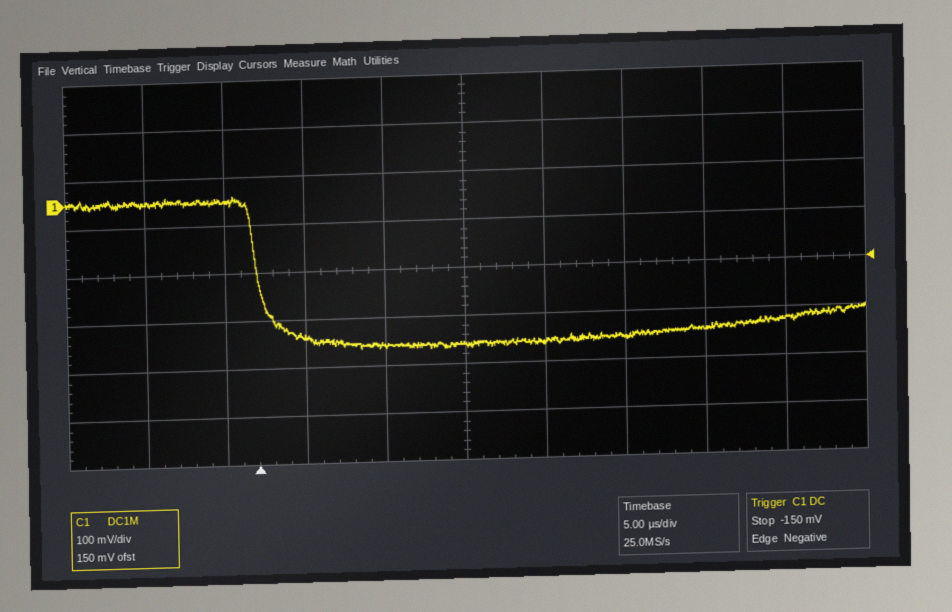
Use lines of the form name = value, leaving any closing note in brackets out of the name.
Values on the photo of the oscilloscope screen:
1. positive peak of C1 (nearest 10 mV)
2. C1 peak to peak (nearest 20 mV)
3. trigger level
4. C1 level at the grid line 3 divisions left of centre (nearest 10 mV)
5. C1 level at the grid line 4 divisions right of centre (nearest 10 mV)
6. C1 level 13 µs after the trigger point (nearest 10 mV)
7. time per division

positive peak of C1 = 10 mV
C1 peak to peak = 320 mV
trigger level = -150 mV
C1 level at the grid line 3 divisions left of centre = 0 mV
C1 level at the grid line 4 divisions right of centre = -270 mV
C1 level 13 µs after the trigger point = -310 mV
time per division = 5 µs
